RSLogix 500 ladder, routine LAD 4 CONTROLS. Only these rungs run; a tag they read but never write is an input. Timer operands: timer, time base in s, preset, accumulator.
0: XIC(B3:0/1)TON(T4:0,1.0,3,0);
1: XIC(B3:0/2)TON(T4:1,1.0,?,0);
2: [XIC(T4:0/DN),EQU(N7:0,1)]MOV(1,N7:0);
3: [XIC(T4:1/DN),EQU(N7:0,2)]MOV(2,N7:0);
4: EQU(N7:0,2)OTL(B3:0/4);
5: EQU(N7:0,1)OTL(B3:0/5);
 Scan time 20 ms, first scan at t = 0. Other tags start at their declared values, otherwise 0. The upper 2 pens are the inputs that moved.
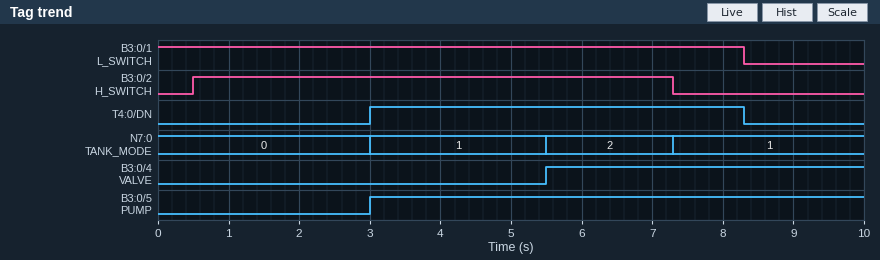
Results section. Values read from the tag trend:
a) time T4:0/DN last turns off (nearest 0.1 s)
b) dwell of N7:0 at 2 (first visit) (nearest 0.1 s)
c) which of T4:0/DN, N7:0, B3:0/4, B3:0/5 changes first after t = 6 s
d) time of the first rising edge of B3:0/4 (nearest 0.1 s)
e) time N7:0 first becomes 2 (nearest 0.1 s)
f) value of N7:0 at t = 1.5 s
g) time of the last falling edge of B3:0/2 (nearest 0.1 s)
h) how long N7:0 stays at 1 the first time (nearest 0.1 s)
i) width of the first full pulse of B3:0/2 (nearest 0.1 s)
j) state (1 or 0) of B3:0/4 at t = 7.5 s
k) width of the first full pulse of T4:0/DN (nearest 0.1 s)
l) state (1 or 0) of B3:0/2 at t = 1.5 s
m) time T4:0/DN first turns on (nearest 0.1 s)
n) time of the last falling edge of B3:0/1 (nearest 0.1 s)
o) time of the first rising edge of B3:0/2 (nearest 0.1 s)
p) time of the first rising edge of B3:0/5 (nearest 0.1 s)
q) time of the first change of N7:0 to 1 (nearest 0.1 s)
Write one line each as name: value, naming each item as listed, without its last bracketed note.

time T4:0/DN last turns off: 8.3 s
dwell of N7:0 at 2 (first visit): 1.8 s
which of T4:0/DN, N7:0, B3:0/4, B3:0/5 changes first after t = 6 s: N7:0
time of the first rising edge of B3:0/4: 5.5 s
time N7:0 first becomes 2: 5.5 s
value of N7:0 at t = 1.5 s: 0
time of the last falling edge of B3:0/2: 7.3 s
how long N7:0 stays at 1 the first time: 2.5 s
width of the first full pulse of B3:0/2: 6.8 s
state (1 or 0) of B3:0/4 at t = 7.5 s: 1
width of the first full pulse of T4:0/DN: 5.3 s
state (1 or 0) of B3:0/2 at t = 1.5 s: 1
time T4:0/DN first turns on: 3.0 s
time of the last falling edge of B3:0/1: 8.3 s
time of the first rising edge of B3:0/2: 0.5 s
time of the first rising edge of B3:0/5: 3.0 s
time of the first change of N7:0 to 1: 3.0 s
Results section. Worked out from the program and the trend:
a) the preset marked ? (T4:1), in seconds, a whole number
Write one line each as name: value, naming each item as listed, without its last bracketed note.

the preset marked ? (T4:1), in seconds, a whole number: 5 s
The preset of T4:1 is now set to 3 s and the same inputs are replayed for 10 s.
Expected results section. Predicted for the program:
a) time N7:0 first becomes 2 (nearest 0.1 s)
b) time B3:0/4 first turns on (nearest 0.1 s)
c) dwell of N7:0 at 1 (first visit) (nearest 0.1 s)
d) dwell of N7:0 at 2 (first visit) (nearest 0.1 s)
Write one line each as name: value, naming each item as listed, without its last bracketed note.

time N7:0 first becomes 2: 3.5 s
time B3:0/4 first turns on: 3.5 s
dwell of N7:0 at 1 (first visit): 0.5 s
dwell of N7:0 at 2 (first visit): 3.8 s
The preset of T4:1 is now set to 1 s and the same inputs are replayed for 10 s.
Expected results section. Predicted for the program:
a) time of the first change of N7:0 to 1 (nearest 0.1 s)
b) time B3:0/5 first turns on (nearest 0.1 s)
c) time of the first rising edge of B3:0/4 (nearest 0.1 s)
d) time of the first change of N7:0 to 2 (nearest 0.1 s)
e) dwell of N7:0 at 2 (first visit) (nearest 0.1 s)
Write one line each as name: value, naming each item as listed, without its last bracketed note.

time of the first change of N7:0 to 1: 7.3 s
time B3:0/5 first turns on: 7.3 s
time of the first rising edge of B3:0/4: 1.5 s
time of the first change of N7:0 to 2: 1.5 s
dwell of N7:0 at 2 (first visit): 5.8 s
